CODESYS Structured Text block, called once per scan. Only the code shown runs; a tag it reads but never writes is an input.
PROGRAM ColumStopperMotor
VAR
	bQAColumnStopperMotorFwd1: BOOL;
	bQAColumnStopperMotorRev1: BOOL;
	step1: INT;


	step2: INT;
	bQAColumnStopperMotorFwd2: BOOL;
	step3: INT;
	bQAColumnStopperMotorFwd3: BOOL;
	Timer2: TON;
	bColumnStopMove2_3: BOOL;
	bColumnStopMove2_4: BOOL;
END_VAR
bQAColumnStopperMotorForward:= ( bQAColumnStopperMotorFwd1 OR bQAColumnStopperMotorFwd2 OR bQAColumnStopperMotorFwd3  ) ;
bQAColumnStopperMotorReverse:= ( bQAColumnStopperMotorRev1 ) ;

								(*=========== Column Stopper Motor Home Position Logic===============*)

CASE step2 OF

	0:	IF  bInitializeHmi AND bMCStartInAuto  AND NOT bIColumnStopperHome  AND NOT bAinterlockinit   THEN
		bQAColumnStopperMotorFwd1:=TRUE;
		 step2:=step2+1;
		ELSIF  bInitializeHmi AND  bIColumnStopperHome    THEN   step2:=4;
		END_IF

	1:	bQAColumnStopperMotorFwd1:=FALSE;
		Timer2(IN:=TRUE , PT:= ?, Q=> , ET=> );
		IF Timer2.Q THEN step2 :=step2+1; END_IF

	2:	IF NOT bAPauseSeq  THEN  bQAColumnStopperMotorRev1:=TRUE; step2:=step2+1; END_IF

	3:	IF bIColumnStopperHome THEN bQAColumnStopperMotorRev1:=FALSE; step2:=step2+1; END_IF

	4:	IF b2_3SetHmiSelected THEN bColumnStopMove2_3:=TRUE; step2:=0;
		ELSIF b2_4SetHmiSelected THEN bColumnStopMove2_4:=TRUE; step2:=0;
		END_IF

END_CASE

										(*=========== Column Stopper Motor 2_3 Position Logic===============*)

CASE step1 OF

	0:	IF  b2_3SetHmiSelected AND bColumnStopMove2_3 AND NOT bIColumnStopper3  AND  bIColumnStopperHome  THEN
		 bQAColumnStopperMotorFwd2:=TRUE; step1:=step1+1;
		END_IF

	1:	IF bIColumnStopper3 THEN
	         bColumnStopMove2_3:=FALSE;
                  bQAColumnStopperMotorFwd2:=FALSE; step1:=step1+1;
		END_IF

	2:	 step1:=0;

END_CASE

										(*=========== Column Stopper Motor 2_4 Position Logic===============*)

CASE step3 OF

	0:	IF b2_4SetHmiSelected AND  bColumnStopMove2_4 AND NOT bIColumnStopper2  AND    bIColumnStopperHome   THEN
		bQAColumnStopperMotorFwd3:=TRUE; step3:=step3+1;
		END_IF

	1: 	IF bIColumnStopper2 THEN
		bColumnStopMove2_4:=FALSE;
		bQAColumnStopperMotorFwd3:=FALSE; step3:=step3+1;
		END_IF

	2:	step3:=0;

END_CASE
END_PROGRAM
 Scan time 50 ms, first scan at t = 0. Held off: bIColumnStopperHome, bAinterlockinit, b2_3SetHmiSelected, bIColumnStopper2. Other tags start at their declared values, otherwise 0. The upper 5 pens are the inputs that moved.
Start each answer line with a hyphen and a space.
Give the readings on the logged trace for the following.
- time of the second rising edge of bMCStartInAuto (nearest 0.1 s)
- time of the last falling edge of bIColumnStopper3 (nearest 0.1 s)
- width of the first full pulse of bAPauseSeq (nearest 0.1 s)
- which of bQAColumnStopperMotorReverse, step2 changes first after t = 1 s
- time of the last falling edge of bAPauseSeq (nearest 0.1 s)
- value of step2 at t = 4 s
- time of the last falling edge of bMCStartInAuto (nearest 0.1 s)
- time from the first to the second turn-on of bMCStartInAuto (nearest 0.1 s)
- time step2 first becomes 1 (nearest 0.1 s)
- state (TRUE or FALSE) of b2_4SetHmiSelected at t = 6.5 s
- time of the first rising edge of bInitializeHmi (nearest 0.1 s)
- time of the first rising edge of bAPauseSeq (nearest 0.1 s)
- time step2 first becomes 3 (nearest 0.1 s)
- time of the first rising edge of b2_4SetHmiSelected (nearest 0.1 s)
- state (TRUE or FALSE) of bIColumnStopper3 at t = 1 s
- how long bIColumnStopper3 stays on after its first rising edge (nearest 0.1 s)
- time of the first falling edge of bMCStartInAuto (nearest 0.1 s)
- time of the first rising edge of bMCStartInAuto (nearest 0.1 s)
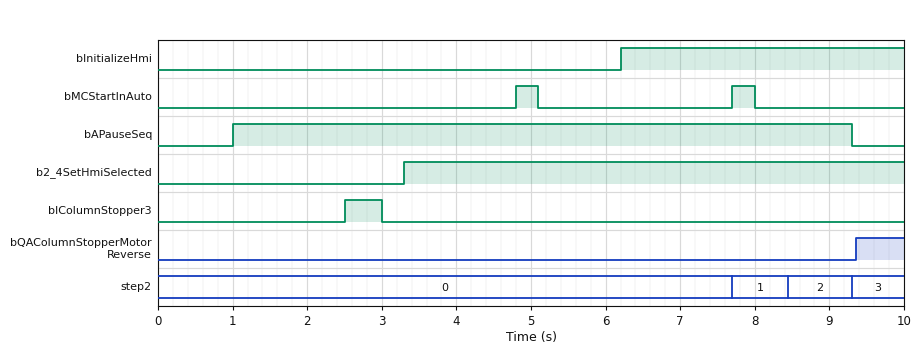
- 7.7 s
- 3.0 s
- 8.3 s
- step2
- 9.3 s
- 0
- 8.0 s
- 2.9 s
- 7.7 s
- TRUE
- 6.2 s
- 1.0 s
- 9.3 s
- 3.3 s
- FALSE
- 0.5 s
- 5.1 s
- 4.8 s
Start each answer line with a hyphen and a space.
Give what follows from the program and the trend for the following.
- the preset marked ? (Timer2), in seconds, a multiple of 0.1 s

- 0.7 s
